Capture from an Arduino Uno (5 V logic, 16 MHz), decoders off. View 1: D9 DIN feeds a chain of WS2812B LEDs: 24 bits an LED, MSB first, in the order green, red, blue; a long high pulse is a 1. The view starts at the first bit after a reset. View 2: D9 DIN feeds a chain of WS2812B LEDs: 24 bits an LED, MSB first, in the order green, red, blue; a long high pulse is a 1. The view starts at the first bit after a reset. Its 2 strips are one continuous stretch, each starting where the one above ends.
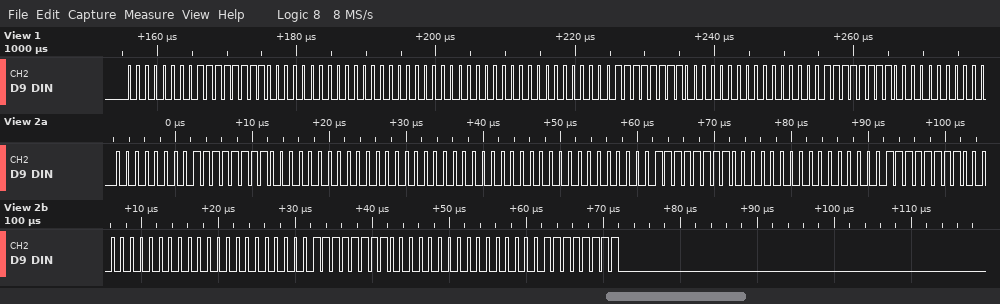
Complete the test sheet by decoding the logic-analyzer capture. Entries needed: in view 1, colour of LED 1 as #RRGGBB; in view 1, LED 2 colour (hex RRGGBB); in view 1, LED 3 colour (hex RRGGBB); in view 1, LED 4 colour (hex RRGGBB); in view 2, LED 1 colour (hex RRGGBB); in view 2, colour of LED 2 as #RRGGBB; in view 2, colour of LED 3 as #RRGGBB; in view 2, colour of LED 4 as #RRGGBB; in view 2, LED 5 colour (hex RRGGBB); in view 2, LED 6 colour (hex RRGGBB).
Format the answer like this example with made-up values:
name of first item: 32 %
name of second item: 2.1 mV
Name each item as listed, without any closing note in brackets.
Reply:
in view 1, colour of LED 1 as #RRGGBB: #FF0000
in view 1, LED 2 colour: #000000
in view 1, LED 3 colour: #FF0000
in view 1, LED 4 colour: #FF0000
in view 2, LED 1 colour: #FF0000
in view 2, colour of LED 2 as #RRGGBB: #000000
in view 2, colour of LED 3 as #RRGGBB: #FF0000
in view 2, colour of LED 4 as #RRGGBB: #FF0000
in view 2, LED 5 colour: #0000FF
in view 2, LED 6 colour: #0000FF
